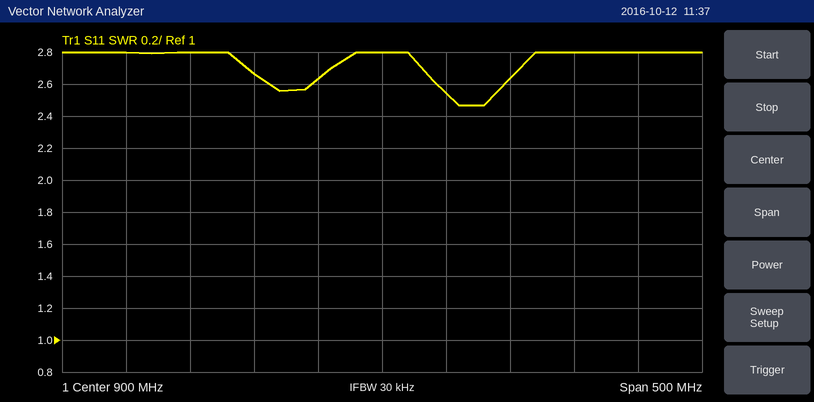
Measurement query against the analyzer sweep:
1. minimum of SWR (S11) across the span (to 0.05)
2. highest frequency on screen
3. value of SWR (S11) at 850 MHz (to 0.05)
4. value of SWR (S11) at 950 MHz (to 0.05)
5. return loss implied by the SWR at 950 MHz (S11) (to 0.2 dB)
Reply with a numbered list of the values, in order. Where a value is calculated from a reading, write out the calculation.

1. 2.45
2. 1.15 GHz
3. 2.65
4. 2.55
5. −20 log10((2.55 − 1)/(2.55 + 1)) ≈ 7.2 dB
